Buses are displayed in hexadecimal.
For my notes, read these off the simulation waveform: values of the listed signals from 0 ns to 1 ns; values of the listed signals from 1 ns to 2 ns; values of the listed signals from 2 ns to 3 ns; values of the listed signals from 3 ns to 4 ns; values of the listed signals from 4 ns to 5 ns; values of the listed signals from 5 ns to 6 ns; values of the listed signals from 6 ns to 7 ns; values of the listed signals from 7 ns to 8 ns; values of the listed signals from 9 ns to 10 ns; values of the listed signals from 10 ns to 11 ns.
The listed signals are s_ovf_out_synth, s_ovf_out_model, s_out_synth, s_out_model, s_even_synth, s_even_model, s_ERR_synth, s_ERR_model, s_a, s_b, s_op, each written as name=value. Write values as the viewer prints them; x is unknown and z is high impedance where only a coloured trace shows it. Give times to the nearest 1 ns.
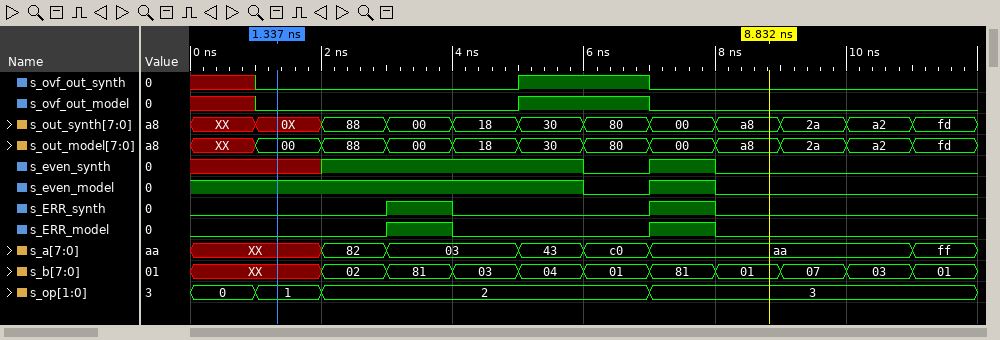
s_ovf_out_synth=x, s_ovf_out_model=x, s_out_synth=XX, s_out_model=XX, s_even_synth=x, s_even_model=1, s_ERR_synth=0, s_ERR_model=0, s_a=XX, s_b=XX, s_op=0
s_ovf_out_synth=0, s_ovf_out_model=0, s_out_synth=0X, s_out_model=00, s_even_synth=x, s_even_model=1, s_ERR_synth=0, s_ERR_model=0, s_a=XX, s_b=XX, s_op=1
s_ovf_out_synth=0, s_ovf_out_model=0, s_out_synth=88, s_out_model=88, s_even_synth=1, s_even_model=1, s_ERR_synth=0, s_ERR_model=0, s_a=82, s_b=02, s_op=2
s_ovf_out_synth=0, s_ovf_out_model=0, s_out_synth=00, s_out_model=00, s_even_synth=1, s_even_model=1, s_ERR_synth=1, s_ERR_model=1, s_a=03, s_b=81, s_op=2
s_ovf_out_synth=0, s_ovf_out_model=0, s_out_synth=18, s_out_model=18, s_even_synth=1, s_even_model=1, s_ERR_synth=0, s_ERR_model=0, s_a=03, s_b=03, s_op=2
s_ovf_out_synth=1, s_ovf_out_model=1, s_out_synth=30, s_out_model=30, s_even_synth=1, s_even_model=1, s_ERR_synth=0, s_ERR_model=0, s_a=43, s_b=04, s_op=2
s_ovf_out_synth=1, s_ovf_out_model=1, s_out_synth=80, s_out_model=80, s_even_synth=0, s_even_model=0, s_ERR_synth=0, s_ERR_model=0, s_a=c0, s_b=01, s_op=2
s_ovf_out_synth=0, s_ovf_out_model=0, s_out_synth=00, s_out_model=00, s_even_synth=1, s_even_model=1, s_ERR_synth=1, s_ERR_model=1, s_a=aa, s_b=81, s_op=3
s_ovf_out_synth=0, s_ovf_out_model=0, s_out_synth=2a, s_out_model=2a, s_even_synth=0, s_even_model=0, s_ERR_synth=0, s_ERR_model=0, s_a=aa, s_b=07, s_op=3
s_ovf_out_synth=0, s_ovf_out_model=0, s_out_synth=a2, s_out_model=a2, s_even_synth=0, s_even_model=0, s_ERR_synth=0, s_ERR_model=0, s_a=aa, s_b=03, s_op=3
